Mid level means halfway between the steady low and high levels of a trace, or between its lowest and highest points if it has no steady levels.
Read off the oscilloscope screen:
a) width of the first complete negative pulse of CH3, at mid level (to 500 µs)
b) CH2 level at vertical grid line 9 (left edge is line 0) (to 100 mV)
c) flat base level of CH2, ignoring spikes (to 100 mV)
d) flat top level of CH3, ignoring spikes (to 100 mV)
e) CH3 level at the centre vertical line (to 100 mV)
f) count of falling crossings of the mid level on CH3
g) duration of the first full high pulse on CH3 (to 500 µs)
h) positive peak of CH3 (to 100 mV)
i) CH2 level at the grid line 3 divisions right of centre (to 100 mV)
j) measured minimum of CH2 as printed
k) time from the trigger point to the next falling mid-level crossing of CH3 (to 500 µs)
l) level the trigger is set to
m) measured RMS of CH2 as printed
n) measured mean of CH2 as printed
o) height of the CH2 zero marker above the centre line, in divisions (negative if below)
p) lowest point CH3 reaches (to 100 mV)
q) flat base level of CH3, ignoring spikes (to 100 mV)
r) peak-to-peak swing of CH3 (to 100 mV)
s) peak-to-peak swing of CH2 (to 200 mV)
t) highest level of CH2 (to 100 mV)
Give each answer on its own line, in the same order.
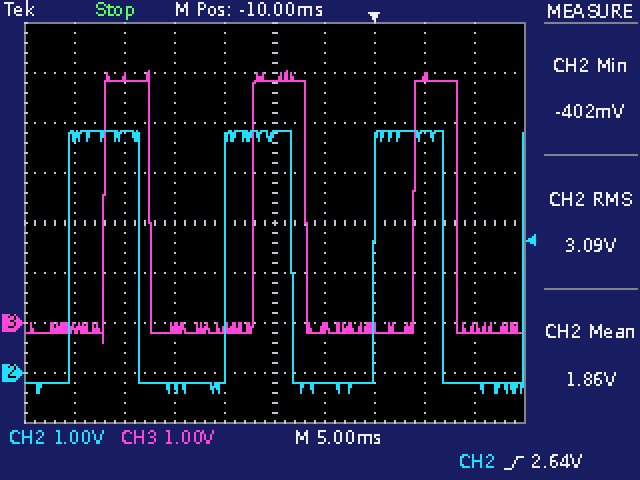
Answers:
10.5 ms
-200 mV
-200 mV
4.8 V
4.8 V
3
4.5 ms
5.0 V
4.8 V
-402 mV
8.5 ms
2.64 V
3.09 V
1.86 V
-3.0 div
-400 mV
-200 mV
5.4 V
5.2 V
4.8 V
